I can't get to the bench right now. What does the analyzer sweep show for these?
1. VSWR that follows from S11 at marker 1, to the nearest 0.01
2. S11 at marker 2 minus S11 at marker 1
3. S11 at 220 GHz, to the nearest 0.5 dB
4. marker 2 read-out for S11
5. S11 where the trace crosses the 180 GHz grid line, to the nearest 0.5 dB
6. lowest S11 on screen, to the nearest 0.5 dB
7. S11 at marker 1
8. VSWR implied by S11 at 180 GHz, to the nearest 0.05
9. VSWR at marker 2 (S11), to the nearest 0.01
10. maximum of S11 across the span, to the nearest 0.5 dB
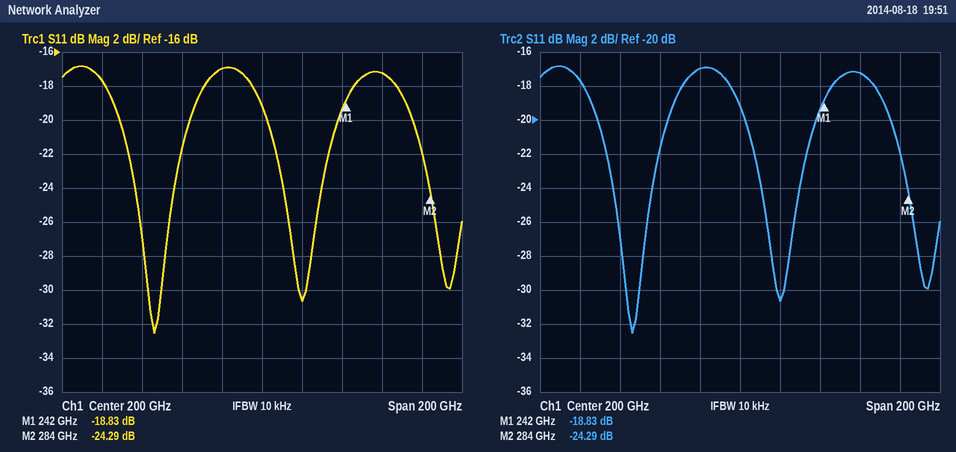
1.26
-5.46 dB
-30.5 dB
-24.29 dB
-17.0 dB
-32.5 dB
-18.83 dB
1.35
1.13
-17.0 dB
